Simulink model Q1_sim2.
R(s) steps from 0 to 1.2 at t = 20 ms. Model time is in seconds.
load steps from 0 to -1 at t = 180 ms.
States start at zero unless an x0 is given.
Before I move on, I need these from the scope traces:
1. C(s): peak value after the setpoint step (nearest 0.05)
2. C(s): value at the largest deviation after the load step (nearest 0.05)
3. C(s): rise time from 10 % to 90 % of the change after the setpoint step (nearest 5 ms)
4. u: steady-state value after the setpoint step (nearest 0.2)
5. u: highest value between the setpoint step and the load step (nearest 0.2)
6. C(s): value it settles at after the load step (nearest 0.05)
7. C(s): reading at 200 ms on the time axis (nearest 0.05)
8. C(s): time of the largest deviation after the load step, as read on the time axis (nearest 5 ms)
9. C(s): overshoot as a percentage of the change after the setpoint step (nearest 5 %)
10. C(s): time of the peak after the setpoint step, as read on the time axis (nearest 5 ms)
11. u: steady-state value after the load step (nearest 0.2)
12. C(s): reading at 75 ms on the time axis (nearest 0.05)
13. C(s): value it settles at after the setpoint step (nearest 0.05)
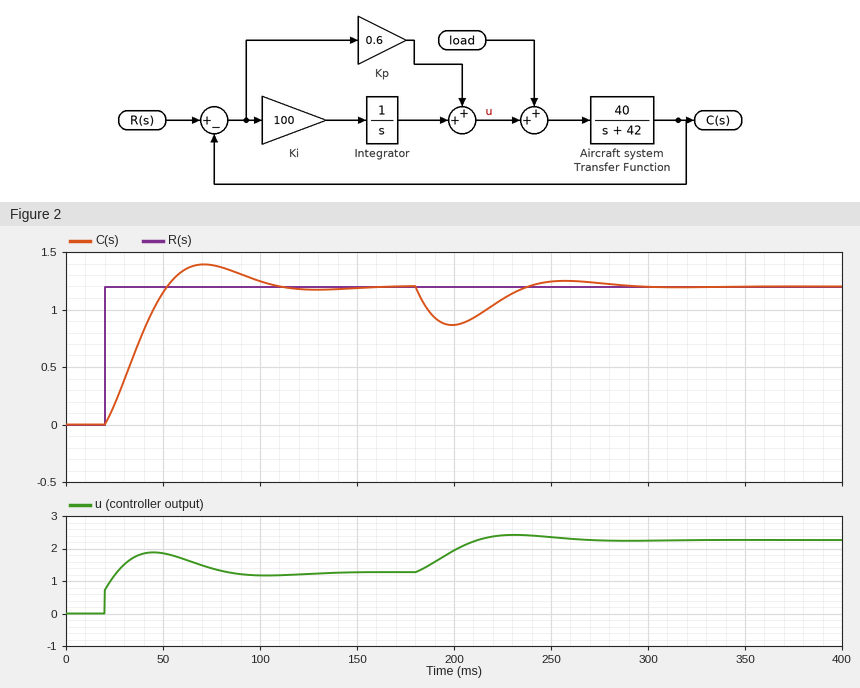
1.40
0.85
25 ms
1.2
1.8
1.20
0.85
200 ms
15 %
70 ms
2.2
1.40
1.20
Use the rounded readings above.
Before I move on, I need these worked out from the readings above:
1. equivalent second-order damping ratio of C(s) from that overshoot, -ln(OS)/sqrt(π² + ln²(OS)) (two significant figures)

0.52
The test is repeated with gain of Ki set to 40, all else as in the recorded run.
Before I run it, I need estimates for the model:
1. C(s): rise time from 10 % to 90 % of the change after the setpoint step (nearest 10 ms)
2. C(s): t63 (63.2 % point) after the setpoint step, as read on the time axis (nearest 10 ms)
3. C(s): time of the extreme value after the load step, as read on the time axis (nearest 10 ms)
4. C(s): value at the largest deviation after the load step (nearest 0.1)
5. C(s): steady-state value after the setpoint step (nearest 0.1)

50 ms
50 ms
210 ms
0.8
1.2
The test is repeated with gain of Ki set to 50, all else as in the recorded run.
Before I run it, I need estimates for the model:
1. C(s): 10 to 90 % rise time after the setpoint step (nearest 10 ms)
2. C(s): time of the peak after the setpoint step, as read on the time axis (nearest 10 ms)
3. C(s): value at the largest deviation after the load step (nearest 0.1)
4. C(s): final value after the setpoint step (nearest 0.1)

40 ms
110 ms
0.8
1.2
